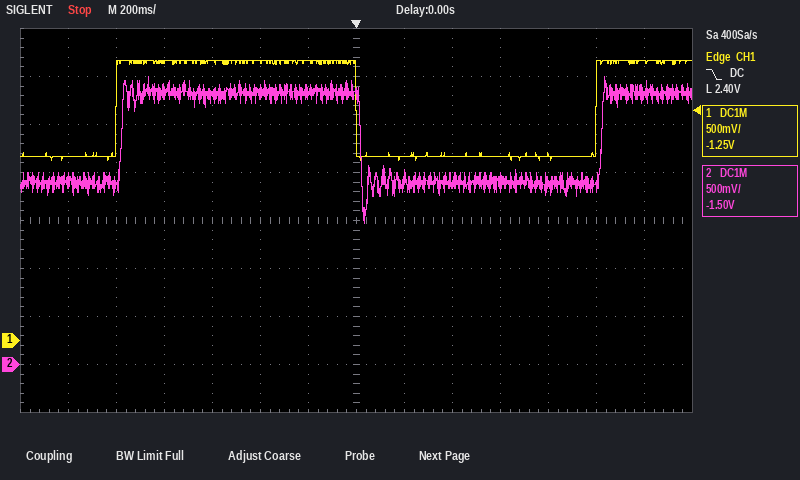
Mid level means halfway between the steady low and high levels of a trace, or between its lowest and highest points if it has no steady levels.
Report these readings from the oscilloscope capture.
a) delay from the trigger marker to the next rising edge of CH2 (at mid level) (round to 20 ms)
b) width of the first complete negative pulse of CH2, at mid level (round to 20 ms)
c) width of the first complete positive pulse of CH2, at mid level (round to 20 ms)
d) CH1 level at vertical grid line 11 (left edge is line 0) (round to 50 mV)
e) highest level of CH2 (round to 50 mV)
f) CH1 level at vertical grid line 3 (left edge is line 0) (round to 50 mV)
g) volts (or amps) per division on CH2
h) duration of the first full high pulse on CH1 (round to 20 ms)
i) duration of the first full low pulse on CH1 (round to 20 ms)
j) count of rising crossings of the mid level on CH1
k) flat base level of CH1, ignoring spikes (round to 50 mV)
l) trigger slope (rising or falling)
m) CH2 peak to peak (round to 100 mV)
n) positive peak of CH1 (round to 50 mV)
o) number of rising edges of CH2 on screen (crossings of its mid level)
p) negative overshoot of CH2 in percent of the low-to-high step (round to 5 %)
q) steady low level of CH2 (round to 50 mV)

1.02 s
1.00 s
1.00 s
1.95 V
3.00 V
2.90 V
500 mV
1.00 s
1.00 s
2
1.90 V
falling
1.50 V
2.90 V
2
45 %
1.90 V
